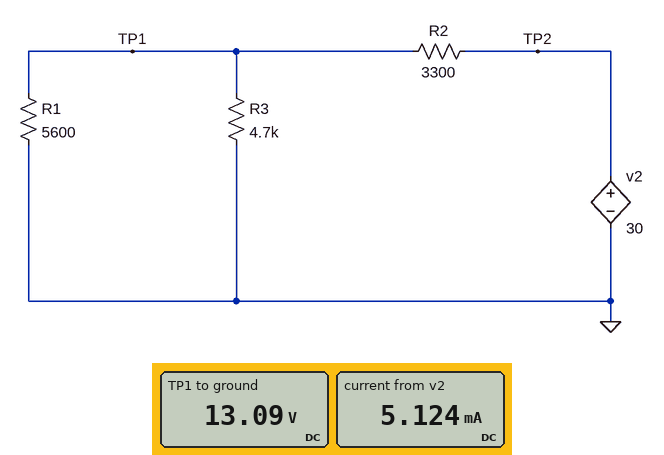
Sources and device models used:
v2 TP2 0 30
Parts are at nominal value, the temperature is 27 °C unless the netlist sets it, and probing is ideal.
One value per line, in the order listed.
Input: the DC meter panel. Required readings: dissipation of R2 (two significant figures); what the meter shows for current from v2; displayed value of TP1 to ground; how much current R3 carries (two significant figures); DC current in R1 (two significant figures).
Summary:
87 mW
5.124 mA
13.09 V
2.8 mA
2.3 mA
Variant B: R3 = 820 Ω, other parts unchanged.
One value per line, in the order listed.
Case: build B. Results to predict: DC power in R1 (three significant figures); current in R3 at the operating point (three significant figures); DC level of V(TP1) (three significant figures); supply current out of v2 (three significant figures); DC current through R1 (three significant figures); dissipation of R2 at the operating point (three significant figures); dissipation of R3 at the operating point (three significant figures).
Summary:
5.10 mW
6.52 mA
5.34 V
7.47 mA
954 µA
184 mW
34.8 mW
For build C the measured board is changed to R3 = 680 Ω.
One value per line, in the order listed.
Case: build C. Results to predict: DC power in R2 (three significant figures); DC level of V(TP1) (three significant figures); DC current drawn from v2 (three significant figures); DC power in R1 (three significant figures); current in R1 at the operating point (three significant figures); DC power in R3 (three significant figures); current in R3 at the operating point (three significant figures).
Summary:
195 mW
4.66 V
7.68 mA
3.87 mW
832 µA
31.9 mW
6.85 mA
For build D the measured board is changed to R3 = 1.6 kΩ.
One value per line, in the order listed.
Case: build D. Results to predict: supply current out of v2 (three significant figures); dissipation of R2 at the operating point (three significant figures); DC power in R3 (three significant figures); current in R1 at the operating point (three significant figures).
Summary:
6.60 mA
144 mW
42.2 mW
1.47 mA
